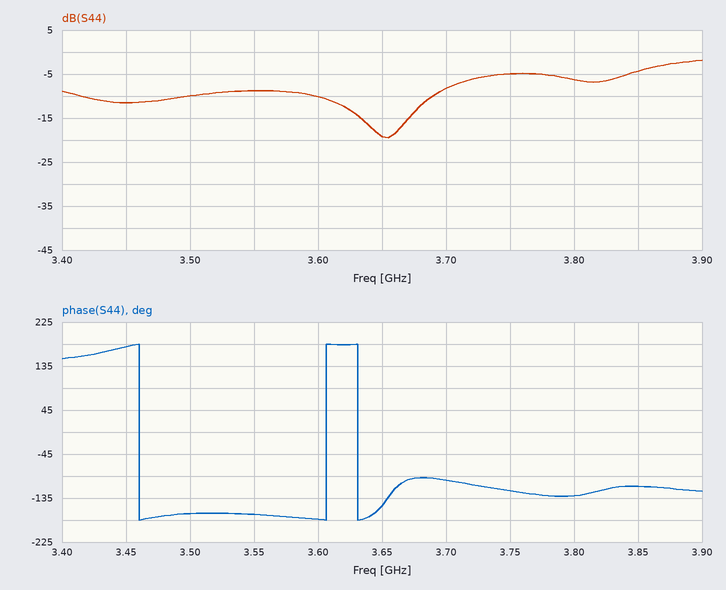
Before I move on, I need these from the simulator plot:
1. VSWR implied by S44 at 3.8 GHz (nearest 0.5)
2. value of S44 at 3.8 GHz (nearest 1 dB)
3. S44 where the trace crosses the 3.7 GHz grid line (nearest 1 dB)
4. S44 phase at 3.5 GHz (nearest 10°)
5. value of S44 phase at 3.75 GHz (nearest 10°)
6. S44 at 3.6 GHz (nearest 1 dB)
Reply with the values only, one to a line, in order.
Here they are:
3.0
-6 dB
-8 dB
-170°
-120°
-10 dB
